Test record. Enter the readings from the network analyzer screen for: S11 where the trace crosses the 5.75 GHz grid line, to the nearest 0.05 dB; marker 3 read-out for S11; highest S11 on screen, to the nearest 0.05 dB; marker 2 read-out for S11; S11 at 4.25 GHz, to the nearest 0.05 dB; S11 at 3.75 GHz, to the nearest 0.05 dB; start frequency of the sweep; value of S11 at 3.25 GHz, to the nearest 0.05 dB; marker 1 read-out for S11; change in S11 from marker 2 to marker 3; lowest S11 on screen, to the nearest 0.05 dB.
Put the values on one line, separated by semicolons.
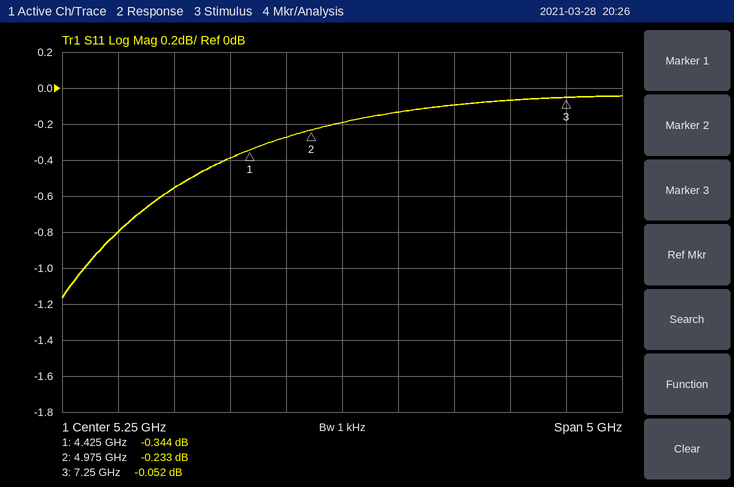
-0.15 dB; -0.052 dB; -0.05 dB; -0.233 dB; -0.40 dB; -0.55 dB; 2.75 GHz; -0.80 dB; -0.344 dB; 0.181 dB; -1.15 dB
